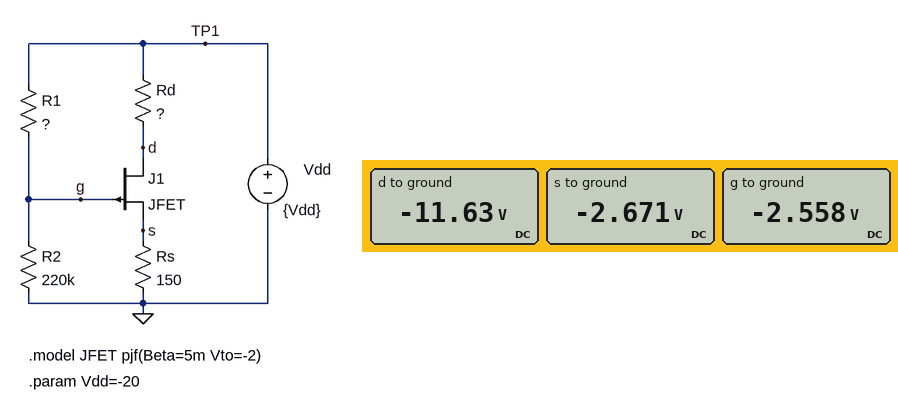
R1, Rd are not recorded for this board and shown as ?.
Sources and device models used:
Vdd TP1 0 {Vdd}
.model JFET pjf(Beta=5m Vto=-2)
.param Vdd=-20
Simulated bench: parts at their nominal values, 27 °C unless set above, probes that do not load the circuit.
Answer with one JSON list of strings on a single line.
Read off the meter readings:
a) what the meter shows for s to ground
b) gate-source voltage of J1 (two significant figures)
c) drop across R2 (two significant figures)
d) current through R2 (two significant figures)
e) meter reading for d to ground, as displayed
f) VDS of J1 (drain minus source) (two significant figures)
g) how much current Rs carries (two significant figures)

["-2.671 V", "110 mV", "2.6 V", "12 µA", "-11.63 V", "-9.0 V", "18 mA"]
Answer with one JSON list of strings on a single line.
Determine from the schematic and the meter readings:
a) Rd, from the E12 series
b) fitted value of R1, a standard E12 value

["470 Ω", "1.5 MΩ"]
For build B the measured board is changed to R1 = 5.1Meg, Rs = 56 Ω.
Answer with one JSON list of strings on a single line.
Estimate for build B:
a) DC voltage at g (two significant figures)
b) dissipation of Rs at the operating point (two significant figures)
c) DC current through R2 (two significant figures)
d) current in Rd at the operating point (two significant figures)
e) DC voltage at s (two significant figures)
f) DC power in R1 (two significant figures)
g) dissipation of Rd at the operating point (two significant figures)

["-830 mV", "17 mW", "3.8 µA", "17 mA", "-970 mV", "72 µW", "140 mW"]
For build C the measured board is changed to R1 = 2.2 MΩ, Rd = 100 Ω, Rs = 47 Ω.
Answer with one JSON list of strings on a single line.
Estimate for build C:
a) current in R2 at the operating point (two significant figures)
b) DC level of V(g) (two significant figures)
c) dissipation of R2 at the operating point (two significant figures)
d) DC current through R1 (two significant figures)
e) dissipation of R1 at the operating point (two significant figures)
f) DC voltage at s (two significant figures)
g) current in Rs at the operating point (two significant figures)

["8.2 µA", "-1.8 V", "15 µW", "8.3 µA", "150 µW", "-1.4 V", "29 mA"]
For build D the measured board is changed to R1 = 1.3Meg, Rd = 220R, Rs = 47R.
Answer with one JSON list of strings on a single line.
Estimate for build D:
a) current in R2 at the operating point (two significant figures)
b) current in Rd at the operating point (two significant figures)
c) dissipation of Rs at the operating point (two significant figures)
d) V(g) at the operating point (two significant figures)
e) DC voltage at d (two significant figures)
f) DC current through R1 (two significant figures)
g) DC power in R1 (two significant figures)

["9.1 µA", "32 mA", "47 mW", "-2.0 V", "-13 V", "14 µA", "250 µW"]
